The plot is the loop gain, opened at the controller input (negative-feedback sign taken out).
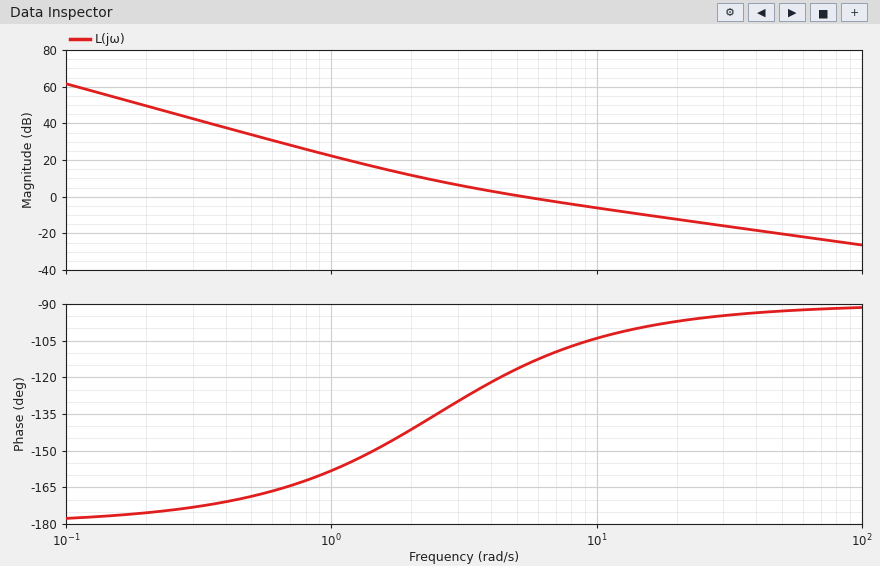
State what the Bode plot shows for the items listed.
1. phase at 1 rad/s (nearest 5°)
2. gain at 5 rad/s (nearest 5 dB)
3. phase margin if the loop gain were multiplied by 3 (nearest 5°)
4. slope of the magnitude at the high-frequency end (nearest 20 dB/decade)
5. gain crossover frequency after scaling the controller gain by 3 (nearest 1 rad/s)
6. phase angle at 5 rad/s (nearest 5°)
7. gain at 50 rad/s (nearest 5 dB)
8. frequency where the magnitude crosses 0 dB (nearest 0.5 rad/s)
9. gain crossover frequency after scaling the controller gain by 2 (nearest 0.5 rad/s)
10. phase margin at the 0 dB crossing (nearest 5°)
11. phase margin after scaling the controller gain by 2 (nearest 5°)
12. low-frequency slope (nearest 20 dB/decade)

-160°
0 dB
80°
-20 dB/decade
15 rad/s
-115°
-20 dB
5.5 rad/s
10.0 rad/s
65°
75°
-40 dB/decade
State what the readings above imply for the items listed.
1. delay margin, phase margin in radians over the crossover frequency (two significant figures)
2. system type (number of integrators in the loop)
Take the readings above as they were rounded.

0.21 s
2
